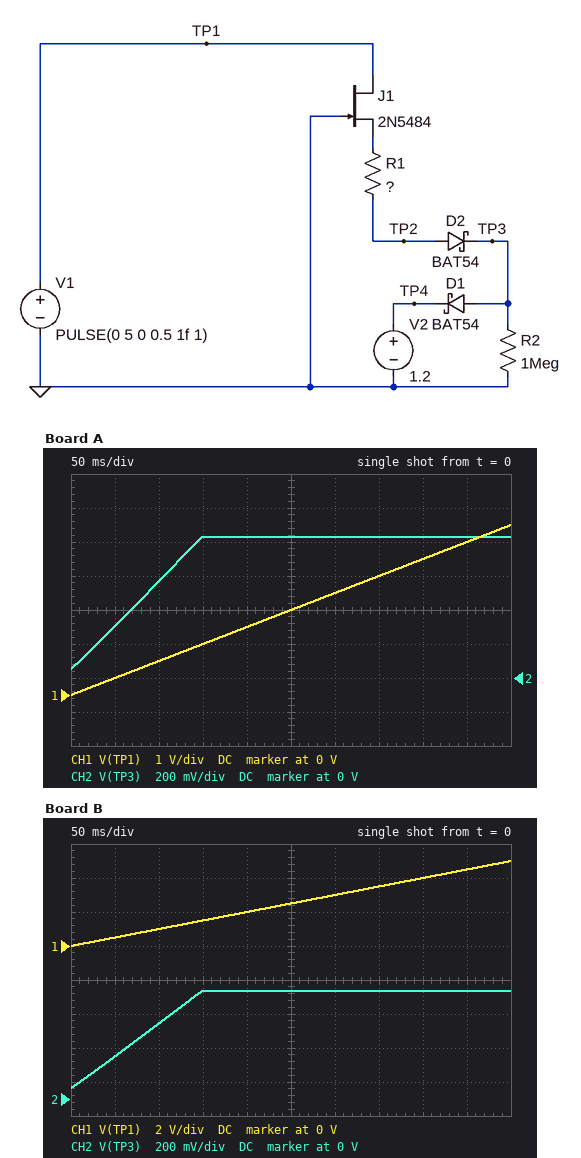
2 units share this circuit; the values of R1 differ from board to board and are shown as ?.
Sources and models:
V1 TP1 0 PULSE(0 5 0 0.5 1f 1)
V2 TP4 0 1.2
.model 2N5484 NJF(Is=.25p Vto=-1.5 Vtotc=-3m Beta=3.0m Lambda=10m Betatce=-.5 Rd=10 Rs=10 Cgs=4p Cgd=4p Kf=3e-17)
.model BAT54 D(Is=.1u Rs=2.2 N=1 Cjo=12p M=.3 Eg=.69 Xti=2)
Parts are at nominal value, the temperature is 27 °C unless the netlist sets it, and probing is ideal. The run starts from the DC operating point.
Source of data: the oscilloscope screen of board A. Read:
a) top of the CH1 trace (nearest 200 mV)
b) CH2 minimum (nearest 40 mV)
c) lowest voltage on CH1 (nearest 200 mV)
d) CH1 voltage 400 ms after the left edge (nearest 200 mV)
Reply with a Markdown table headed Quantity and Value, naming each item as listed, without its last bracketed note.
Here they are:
| Quantity | Value |
|---|---|
| top of the CH1 trace | 5.0 V |
| CH2 minimum | 40 mV |
| lowest voltage on CH1 | 0 V |
| CH1 voltage 400 ms after the left edge | 4.0 V |
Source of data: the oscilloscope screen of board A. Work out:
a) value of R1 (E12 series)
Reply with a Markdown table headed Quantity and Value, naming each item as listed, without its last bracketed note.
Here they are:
| Quantity | Value |
|---|---|
| value of R1 | 820 kΩ |
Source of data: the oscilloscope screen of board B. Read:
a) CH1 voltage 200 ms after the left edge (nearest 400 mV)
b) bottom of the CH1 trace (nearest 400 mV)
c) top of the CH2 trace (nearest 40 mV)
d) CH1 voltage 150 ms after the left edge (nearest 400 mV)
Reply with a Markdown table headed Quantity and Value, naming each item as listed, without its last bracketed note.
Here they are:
| Quantity | Value |
|---|---|
| CH1 voltage 200 ms after the left edge | 2.0 V |
| bottom of the CH1 trace | 0 V |
| top of the CH2 trace | 640 mV |
| CH1 voltage 150 ms after the left edge | 1.6 V |
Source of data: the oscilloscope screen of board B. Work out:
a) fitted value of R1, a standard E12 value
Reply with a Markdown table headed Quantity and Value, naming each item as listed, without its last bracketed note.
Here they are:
| Quantity | Value |
|---|---|
| fitted value of R1, a standard E12 value | 1.5 MΩ |
